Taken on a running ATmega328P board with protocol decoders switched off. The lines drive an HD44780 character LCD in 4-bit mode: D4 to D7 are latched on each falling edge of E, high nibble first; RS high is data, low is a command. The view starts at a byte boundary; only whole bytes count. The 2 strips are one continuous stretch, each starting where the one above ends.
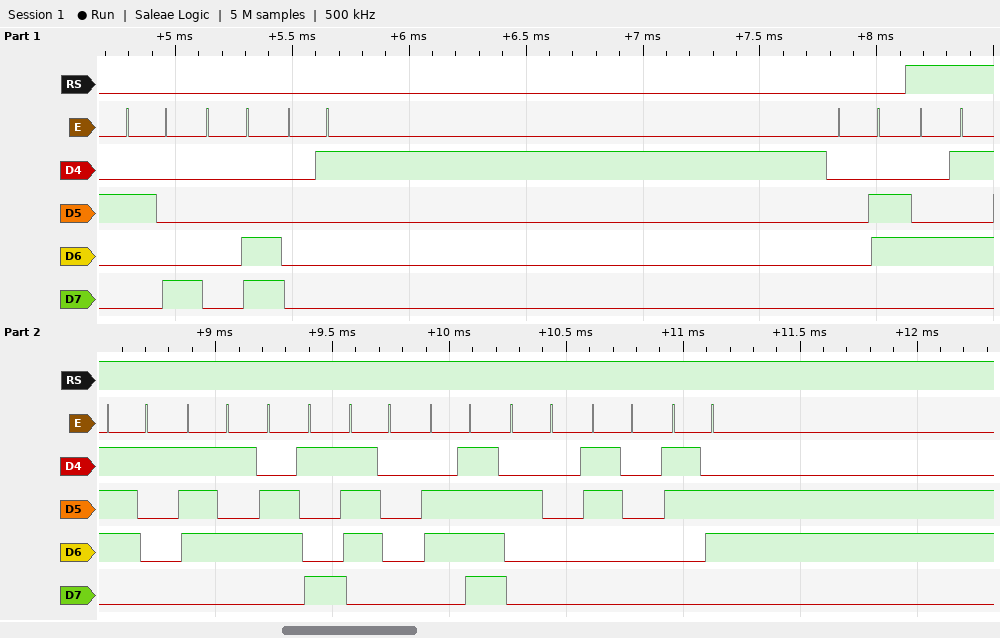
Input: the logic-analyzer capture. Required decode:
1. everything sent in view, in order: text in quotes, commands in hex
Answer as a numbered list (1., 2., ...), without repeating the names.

1. 0x28 0x0C 0x01 0x06 "Equipo 06"
